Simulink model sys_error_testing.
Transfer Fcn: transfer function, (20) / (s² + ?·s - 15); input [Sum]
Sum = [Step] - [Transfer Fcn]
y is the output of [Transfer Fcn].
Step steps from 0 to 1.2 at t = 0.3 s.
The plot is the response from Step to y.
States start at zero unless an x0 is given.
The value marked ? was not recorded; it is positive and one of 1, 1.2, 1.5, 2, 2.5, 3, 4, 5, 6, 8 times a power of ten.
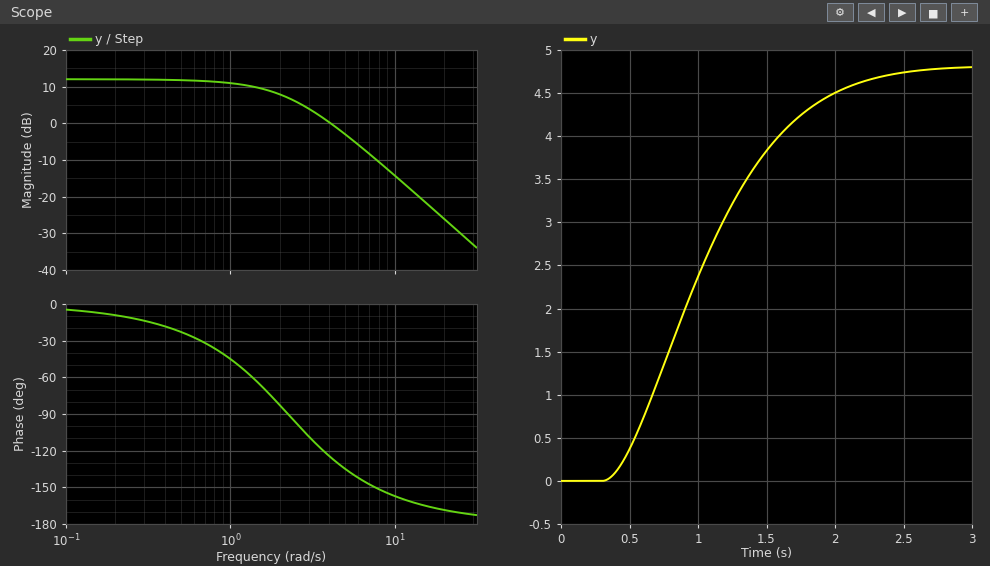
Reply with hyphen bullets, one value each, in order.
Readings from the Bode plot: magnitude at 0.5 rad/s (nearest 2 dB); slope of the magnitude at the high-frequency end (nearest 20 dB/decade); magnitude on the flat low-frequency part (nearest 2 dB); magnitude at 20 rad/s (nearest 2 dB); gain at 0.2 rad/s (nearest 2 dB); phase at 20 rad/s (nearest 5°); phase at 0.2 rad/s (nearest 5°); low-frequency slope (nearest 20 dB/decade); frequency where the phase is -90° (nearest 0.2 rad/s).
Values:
- 12 dB
- -40 dB/decade
- 12 dB
- -26 dB
- 12 dB
- -170°
- -10°
- 0 dB/decade
- 2.2 rad/s
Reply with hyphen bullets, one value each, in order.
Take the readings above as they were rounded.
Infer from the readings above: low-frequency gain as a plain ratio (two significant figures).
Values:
- 4.0
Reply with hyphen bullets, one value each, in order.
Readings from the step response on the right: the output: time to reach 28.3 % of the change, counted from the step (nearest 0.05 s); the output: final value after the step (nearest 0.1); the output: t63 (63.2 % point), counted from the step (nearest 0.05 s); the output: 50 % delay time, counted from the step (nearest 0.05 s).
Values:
- 0.45 s
- 4.8
- 0.90 s
- 0.70 s
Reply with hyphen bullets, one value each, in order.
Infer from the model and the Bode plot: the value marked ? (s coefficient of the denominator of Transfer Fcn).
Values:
- 4
